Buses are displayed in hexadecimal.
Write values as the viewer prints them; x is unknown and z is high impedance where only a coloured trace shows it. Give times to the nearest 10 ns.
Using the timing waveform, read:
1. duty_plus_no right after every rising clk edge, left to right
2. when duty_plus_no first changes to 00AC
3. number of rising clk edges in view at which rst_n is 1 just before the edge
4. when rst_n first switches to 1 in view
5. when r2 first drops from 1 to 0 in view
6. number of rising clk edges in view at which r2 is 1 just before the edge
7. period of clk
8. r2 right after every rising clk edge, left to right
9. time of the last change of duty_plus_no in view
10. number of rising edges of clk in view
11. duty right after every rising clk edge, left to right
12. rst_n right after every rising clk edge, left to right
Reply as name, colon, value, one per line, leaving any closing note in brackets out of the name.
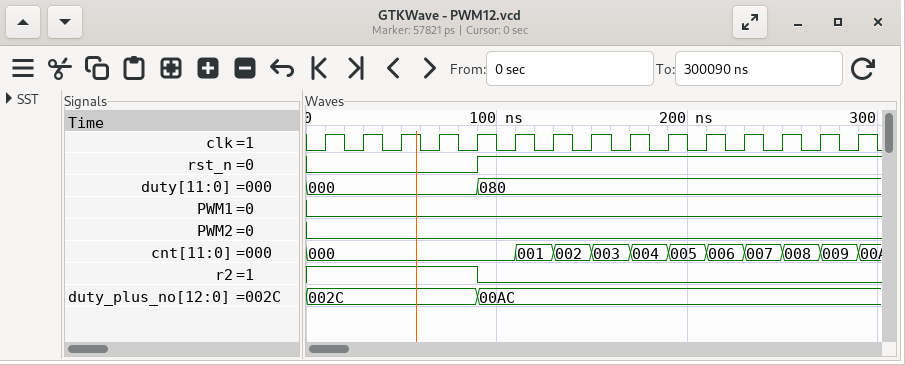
duty_plus_no right after every rising clk edge, left to right: 002C, 002C, 002C, 002C, 00AC, 00AC, 00AC, 00AC, 00AC, 00AC, 00AC, 00AC, 00AC, 00AC, 00AC
when duty_plus_no first changes to 00AC: 90 ns
number of rising clk edges in view at which rst_n is 1 just before the edge: 10
when rst_n first switches to 1 in view: 90 ns
when r2 first drops from 1 to 0 in view: 90 ns
number of rising clk edges in view at which r2 is 1 just before the edge: 5
period of clk: 20 ns
r2 right after every rising clk edge, left to right: 1 1 1 1 0 0 0 0 0 0 0 0 0 0 0
time of the last change of duty_plus_no in view: 90 ns
number of rising edges of clk in view: 15
duty right after every rising clk edge, left to right: 000, 000, 000, 000, 080, 080, 080, 080, 080, 080, 080, 080, 080, 080, 080
rst_n right after every rising clk edge, left to right: 0 0 0 0 1 1 1 1 1 1 1 1 1 1 1
